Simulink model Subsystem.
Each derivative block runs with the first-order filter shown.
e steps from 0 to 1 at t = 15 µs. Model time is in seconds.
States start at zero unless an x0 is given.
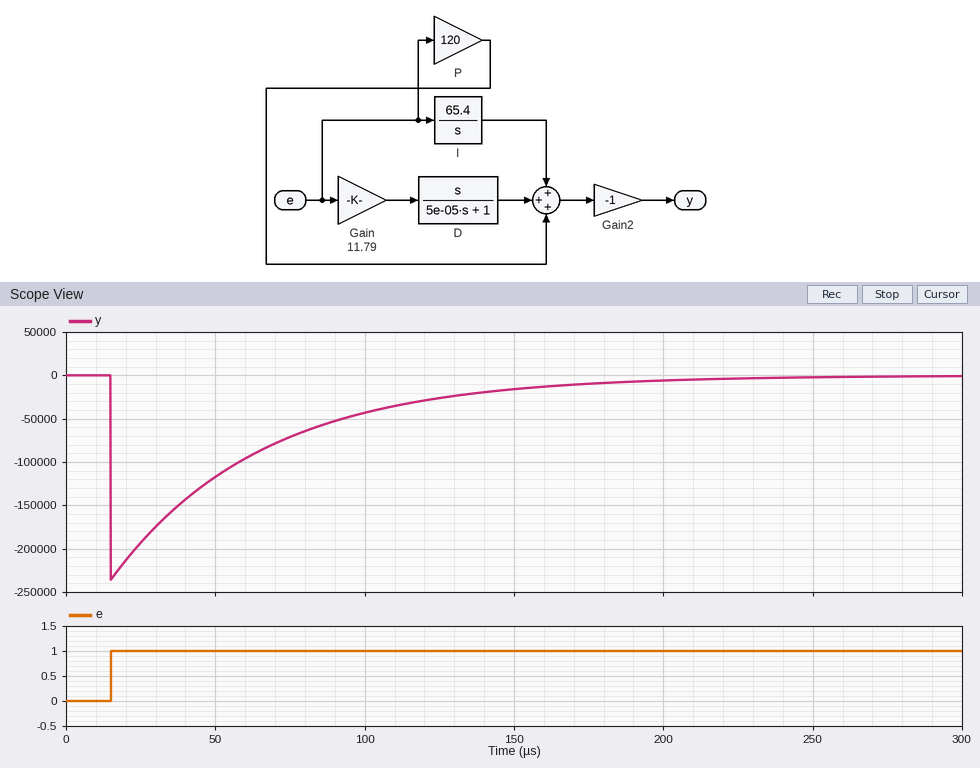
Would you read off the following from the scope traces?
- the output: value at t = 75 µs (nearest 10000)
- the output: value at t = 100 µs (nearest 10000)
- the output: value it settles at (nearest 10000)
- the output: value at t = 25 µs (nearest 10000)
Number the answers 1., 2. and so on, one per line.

1. -70000
2. -40000
3. 0
4. -190000
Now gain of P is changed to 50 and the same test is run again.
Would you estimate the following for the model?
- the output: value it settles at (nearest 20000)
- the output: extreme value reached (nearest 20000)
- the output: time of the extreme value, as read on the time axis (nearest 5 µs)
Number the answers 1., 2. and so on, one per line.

1. 0
2. -240000
3. 15 µs
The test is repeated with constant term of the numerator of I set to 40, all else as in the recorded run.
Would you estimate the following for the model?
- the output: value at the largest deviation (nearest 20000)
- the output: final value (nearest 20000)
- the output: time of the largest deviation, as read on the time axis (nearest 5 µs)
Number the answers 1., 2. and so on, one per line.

1. -240000
2. 0
3. 15 µs
